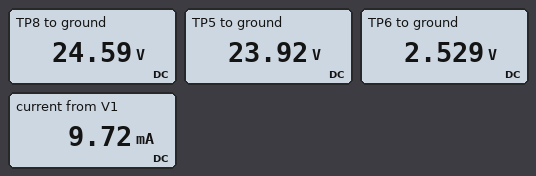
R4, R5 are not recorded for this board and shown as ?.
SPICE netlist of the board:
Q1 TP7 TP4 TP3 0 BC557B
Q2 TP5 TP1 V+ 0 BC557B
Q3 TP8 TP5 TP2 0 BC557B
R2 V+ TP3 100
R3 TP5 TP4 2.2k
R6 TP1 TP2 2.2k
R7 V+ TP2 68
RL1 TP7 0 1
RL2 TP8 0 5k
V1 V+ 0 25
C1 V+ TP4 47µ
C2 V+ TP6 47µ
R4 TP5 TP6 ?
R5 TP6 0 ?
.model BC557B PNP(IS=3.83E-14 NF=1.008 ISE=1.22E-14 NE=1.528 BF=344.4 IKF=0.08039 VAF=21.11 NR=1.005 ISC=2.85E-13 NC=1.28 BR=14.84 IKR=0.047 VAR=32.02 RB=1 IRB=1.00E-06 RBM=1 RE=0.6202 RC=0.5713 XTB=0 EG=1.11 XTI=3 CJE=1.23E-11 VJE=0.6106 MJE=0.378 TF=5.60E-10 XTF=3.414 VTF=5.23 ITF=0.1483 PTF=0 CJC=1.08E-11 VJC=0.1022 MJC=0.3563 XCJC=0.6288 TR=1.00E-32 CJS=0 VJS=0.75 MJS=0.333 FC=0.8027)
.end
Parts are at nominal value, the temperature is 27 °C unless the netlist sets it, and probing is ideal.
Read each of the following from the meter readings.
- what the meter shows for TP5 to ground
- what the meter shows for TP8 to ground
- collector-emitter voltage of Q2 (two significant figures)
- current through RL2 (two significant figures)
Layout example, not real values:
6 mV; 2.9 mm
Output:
23.92 V; 24.59 V; -1.1 V; 4.9 mA
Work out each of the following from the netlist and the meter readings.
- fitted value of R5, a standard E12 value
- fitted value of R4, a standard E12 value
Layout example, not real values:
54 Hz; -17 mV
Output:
3.9 kΩ; 33 kΩ
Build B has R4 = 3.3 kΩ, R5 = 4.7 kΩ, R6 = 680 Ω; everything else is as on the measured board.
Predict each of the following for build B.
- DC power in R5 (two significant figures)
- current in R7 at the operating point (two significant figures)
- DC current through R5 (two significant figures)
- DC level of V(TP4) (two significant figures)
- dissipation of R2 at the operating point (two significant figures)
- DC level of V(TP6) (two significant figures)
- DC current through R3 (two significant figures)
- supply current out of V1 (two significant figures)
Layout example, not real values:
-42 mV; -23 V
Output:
41 mW; 7.8 mA; 3.0 mA; 24 V; 3.5 mW; 14 V; 8.6 µA; 14 mA
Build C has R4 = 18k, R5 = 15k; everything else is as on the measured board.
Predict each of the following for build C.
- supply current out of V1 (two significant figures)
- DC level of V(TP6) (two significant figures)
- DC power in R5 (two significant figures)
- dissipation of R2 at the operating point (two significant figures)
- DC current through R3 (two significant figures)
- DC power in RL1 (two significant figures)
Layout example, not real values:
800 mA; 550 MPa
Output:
9.9 mA; 11 V; 7.9 mW; 1.8 mW; 6.1 µA; 18 µW
